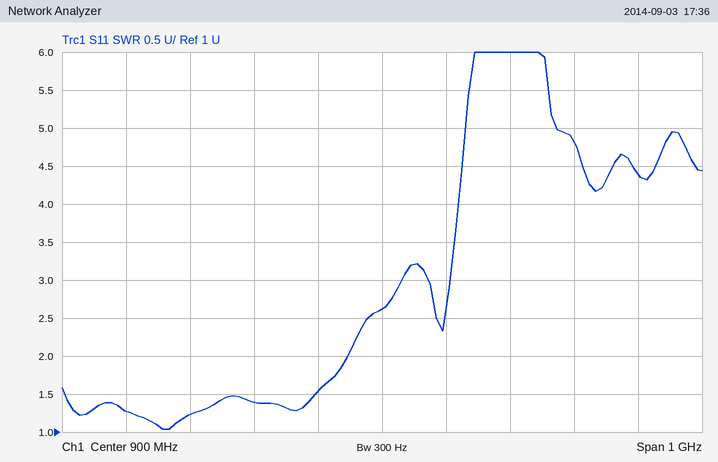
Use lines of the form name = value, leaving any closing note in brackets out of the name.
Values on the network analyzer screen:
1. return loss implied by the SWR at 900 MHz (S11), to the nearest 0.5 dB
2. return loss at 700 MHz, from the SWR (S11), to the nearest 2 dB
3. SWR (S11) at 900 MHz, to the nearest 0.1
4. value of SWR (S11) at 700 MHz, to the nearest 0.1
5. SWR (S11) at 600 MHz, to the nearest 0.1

return loss implied by the SWR at 900 MHz (S11), to the nearest 0.5 dB = 7.0 dB
return loss at 700 MHz, from the SWR (S11), to the nearest 2 dB = 16 dB
SWR (S11) at 900 MHz, to the nearest 0.1 = 2.6
value of SWR (S11) at 700 MHz, to the nearest 0.1 = 1.4
SWR (S11) at 600 MHz, to the nearest 0.1 = 1.2
